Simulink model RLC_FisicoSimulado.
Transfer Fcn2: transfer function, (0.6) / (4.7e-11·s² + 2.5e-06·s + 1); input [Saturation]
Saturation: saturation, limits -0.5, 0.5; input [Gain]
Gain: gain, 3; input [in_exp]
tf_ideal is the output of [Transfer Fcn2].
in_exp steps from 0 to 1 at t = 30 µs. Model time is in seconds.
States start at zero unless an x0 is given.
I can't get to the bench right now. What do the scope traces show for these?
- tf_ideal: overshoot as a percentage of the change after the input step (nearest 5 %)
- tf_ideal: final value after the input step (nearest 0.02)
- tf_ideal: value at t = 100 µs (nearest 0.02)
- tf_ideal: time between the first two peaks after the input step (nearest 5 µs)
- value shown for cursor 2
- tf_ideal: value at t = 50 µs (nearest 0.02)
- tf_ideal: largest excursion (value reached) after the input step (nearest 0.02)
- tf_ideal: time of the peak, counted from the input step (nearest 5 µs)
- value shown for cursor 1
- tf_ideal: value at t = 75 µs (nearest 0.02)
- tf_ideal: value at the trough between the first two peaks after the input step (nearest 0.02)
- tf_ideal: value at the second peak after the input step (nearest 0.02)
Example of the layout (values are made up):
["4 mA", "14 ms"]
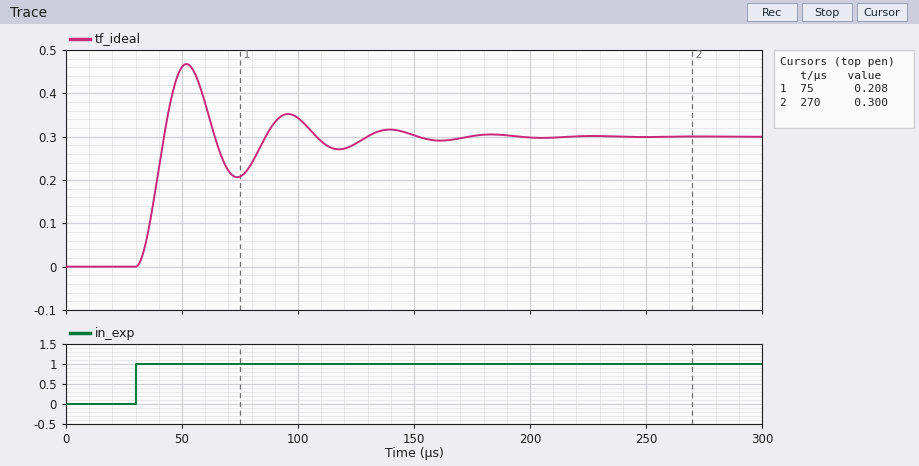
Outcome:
["55 %", "0.30", "0.34", "45 µs", "0.300", "0.46", "0.46", "20 µs", "0.208", "0.20", "0.20", "0.36"]
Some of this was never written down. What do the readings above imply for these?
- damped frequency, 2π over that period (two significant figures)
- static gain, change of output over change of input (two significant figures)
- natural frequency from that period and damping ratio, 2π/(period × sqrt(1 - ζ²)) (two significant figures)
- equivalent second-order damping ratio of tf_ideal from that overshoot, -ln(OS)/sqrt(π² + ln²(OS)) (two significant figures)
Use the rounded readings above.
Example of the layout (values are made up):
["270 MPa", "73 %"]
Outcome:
["0.14 rad/µs", "0.30", "0.14 rad/µs", "0.19"]
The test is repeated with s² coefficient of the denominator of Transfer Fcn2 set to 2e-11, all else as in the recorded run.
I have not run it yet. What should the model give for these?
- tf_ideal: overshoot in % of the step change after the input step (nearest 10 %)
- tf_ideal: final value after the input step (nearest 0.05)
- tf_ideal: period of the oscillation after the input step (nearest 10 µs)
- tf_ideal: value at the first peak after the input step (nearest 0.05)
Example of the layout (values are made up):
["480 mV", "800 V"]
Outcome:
["40 %", "0.30", "30 µs", "0.40"]
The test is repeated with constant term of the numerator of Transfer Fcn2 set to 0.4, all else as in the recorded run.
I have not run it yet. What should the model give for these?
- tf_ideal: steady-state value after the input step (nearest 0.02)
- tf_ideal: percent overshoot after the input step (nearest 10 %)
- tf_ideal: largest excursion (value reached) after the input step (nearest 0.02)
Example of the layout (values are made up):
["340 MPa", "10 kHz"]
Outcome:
["0.20", "60 %", "0.32"]
